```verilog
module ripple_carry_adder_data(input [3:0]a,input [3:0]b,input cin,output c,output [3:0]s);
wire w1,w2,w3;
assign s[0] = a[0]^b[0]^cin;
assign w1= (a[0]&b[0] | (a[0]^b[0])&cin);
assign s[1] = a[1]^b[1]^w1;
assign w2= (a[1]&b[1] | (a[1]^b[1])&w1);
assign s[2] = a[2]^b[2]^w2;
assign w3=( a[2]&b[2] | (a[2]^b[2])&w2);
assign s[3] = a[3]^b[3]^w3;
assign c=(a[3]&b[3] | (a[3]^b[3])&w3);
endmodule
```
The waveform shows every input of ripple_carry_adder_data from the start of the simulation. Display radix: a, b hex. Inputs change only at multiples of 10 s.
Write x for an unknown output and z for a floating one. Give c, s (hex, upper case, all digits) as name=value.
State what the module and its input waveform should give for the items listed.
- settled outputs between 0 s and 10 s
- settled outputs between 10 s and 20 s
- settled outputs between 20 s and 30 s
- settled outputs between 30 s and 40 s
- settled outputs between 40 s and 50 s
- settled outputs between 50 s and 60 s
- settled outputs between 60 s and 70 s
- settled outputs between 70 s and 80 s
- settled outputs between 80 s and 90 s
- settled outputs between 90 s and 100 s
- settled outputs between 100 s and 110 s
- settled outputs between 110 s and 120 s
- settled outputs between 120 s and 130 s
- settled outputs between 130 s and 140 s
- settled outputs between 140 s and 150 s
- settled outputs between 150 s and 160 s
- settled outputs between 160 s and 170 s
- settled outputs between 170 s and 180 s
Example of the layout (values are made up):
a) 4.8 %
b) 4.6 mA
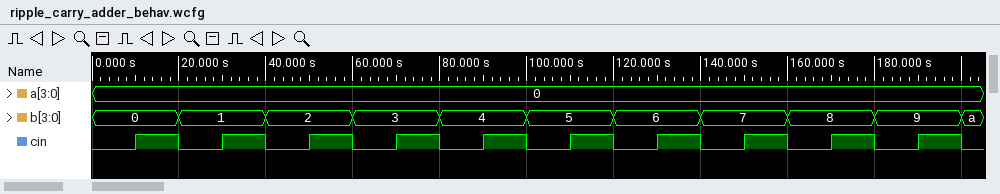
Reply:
a) c=0, s=0
b) c=0, s=1
c) c=0, s=1
d) c=0, s=2
e) c=0, s=2
f) c=0, s=3
g) c=0, s=3
h) c=0, s=4
i) c=0, s=4
j) c=0, s=5
k) c=0, s=5
l) c=0, s=6
m) c=0, s=6
n) c=0, s=7
o) c=0, s=7
p) c=0, s=8
q) c=0, s=8
r) c=0, s=9
